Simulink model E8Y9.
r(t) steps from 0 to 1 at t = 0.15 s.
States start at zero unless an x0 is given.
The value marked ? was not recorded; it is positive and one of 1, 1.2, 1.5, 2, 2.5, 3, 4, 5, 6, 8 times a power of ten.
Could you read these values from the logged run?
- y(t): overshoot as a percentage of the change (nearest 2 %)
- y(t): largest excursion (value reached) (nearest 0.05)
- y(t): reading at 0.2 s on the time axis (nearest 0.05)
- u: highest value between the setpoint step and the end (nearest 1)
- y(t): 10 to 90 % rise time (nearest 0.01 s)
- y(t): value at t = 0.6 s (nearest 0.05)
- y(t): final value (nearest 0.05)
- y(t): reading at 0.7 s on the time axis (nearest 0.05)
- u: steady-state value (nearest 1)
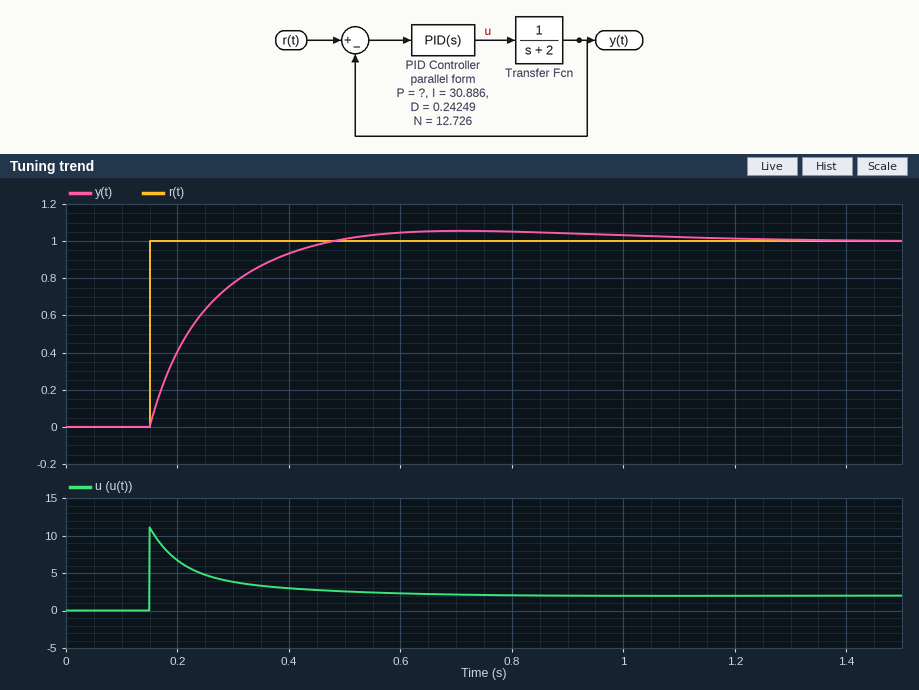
6 %
1.05
0.40
11
0.21 s
1.05
1.00
1.05
2
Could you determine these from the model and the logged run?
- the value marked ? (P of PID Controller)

8
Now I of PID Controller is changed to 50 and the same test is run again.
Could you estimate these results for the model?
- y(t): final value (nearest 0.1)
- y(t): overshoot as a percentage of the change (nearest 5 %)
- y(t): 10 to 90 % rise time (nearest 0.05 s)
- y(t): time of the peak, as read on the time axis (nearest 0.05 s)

1.0
10 %
0.15 s
0.55 s
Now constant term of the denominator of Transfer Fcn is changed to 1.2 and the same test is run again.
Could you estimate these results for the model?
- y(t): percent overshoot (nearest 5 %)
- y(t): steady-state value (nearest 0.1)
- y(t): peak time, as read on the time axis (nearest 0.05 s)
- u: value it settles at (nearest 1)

10 %
1.0
0.65 s
1
